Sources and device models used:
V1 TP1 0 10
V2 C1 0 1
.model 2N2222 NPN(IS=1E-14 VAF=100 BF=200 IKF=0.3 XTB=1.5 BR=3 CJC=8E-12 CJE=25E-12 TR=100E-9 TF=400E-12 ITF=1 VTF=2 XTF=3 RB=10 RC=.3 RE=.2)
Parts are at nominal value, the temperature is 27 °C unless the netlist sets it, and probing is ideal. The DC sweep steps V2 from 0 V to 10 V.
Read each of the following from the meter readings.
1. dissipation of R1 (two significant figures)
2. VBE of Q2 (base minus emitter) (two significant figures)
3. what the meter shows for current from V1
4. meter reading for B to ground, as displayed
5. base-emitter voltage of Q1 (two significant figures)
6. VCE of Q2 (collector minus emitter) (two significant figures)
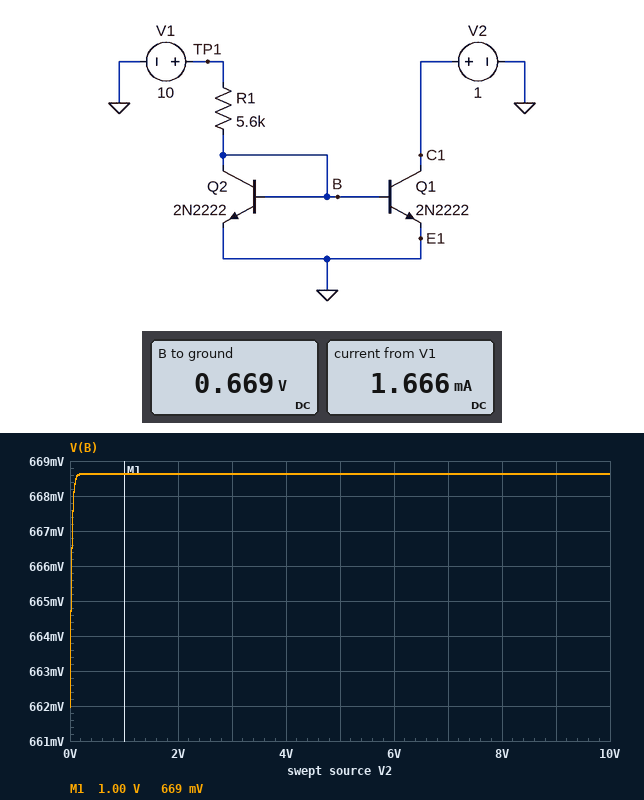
16 mW
670 mV
1.666 mA
0.669 V
670 mV
670 mV
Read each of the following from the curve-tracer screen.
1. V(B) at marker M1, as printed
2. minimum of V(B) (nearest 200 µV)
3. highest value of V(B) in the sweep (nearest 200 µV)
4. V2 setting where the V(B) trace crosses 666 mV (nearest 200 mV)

669 mV
662.0 mV
668.6 mV
0 V
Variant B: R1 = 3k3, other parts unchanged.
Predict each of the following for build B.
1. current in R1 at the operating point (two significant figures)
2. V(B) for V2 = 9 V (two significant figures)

2.8 mA
680 mV
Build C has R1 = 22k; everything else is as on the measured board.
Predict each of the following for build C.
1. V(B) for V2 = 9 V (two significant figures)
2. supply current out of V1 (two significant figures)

630 mV
430 µA
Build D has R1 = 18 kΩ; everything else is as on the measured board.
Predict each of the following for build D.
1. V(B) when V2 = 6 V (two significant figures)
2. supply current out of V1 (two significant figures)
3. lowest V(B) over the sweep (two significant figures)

640 mV
520 µA
630 mV
